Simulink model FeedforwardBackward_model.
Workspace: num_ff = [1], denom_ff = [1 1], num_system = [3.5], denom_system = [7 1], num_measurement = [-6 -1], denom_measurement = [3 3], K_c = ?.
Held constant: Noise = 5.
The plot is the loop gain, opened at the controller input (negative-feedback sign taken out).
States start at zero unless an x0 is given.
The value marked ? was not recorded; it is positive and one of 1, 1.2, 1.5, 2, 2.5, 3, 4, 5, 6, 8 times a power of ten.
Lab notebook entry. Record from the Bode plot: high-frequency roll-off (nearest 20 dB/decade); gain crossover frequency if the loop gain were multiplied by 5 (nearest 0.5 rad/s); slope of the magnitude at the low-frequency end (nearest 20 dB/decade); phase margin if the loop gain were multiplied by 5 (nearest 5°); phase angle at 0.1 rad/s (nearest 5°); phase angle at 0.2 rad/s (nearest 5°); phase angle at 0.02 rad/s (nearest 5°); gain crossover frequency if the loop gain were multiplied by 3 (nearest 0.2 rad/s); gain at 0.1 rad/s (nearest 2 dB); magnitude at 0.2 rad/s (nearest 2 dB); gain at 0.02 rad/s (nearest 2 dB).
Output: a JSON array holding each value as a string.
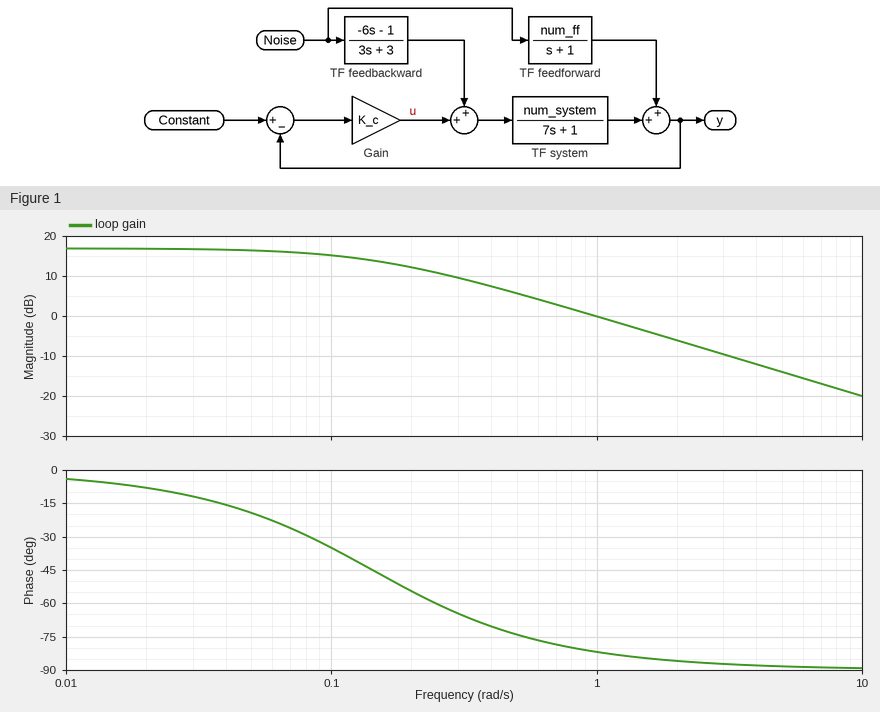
["-20 dB/decade", "5.0 rad/s", "0 dB/decade", "90°", "-35°", "-55°", "-10°", "3.0 rad/s", "16 dB", "12 dB", "16 dB"]
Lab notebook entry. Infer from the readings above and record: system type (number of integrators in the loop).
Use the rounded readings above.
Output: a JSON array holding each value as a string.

["0"]
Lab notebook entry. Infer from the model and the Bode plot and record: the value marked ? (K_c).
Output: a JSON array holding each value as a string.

["2"]
